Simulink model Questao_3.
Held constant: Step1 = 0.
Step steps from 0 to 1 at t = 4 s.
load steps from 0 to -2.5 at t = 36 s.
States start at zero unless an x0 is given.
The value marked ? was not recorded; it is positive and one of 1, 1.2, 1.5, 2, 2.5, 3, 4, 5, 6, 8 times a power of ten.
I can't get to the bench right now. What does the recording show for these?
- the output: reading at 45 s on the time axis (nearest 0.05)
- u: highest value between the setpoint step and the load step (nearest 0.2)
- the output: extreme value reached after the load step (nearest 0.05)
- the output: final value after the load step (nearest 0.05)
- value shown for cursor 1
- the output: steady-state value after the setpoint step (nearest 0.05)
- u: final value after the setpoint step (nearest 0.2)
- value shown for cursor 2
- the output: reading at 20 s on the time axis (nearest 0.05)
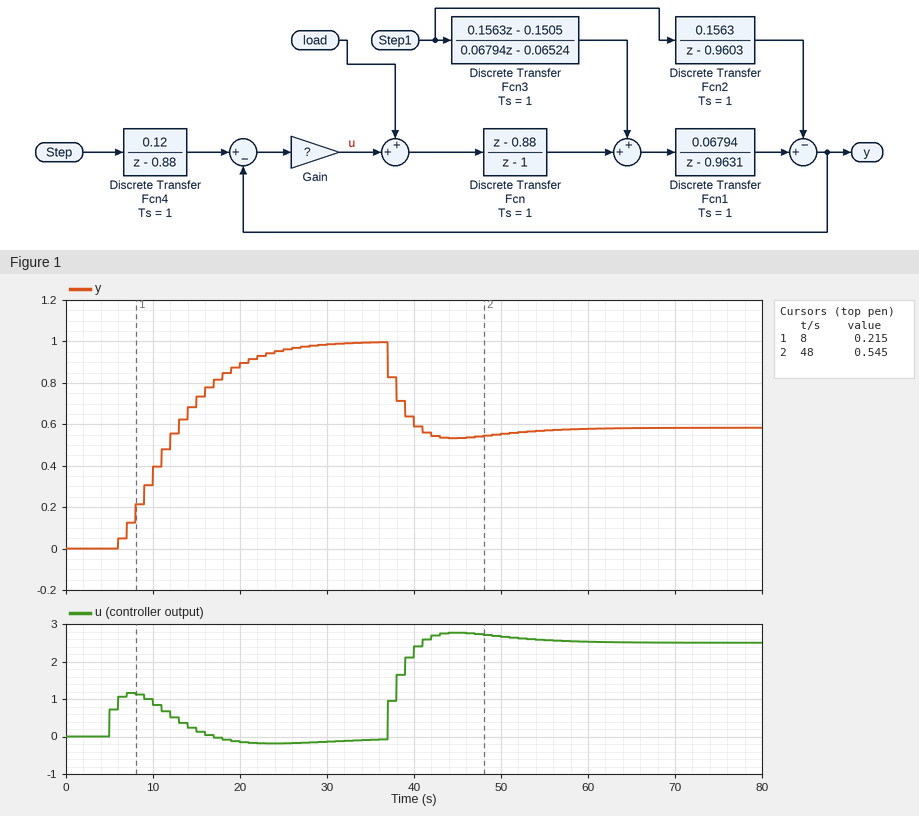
0.55
1.2
0.55
0.60
0.215
1.00
0.0
0.545
0.90
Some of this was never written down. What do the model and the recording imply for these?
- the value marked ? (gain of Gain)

6
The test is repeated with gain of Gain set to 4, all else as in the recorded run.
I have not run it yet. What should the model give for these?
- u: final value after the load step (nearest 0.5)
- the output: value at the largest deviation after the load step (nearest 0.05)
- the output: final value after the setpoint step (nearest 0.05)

2.5
0.30
1.00
